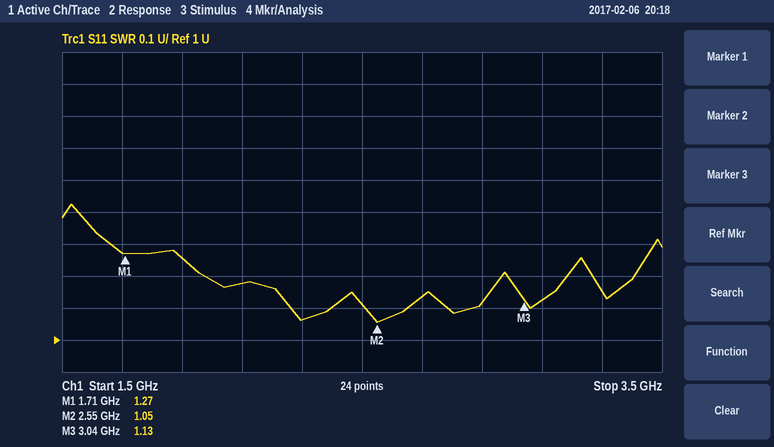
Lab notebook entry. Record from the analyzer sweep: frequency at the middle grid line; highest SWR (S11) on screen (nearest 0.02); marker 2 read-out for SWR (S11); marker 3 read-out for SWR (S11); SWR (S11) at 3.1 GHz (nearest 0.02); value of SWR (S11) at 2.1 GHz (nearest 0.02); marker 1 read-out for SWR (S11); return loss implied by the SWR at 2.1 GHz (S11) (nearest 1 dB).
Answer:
2.5 GHz
1.42
1.05
1.13
1.12
1.18
1.27
22 dB
